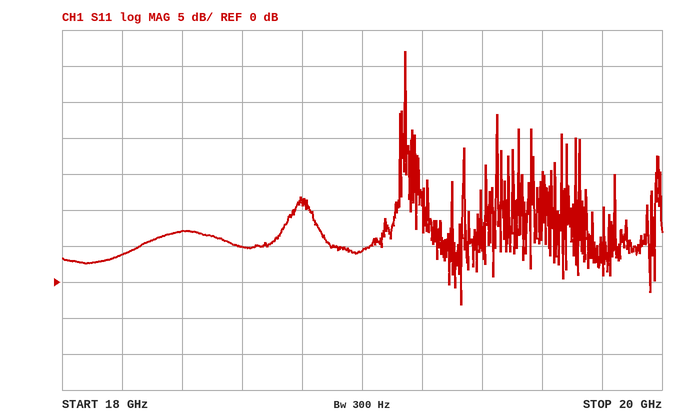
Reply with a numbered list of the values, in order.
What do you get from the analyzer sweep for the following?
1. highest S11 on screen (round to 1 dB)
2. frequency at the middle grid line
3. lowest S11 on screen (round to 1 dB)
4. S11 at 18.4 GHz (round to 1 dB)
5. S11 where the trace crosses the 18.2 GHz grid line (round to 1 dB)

1. 32 dB
2. 19 GHz
3. -3 dB
4. 7 dB
5. 4 dB
